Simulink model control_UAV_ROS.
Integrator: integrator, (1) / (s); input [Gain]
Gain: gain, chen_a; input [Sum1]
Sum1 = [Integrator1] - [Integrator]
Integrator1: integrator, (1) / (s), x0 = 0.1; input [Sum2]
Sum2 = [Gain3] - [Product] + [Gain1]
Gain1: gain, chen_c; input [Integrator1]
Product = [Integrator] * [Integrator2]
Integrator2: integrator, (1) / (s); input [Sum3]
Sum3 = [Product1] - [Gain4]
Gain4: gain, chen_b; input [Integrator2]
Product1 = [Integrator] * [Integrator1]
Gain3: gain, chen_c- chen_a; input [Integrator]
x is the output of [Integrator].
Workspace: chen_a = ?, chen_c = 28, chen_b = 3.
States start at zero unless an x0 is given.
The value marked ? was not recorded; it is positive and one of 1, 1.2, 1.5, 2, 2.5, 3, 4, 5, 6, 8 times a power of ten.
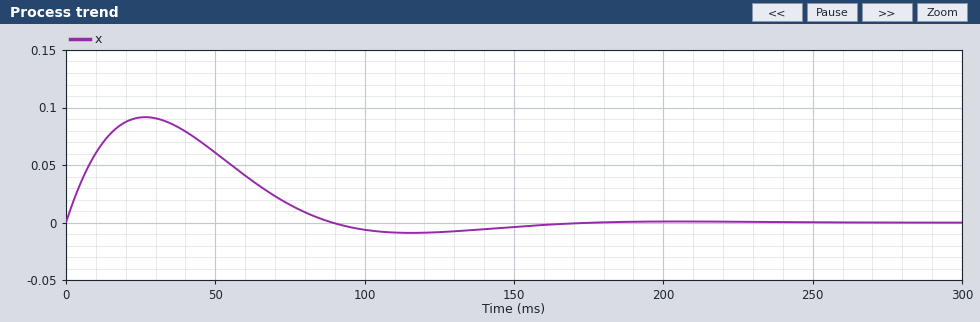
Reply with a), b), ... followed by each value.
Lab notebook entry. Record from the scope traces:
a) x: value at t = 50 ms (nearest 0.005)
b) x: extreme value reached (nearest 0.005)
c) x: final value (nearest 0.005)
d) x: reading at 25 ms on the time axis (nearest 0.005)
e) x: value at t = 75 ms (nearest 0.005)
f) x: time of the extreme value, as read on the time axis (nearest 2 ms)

a) 0.060
b) 0.090
c) 0.000
d) 0.090
e) 0.015
f) 26 ms
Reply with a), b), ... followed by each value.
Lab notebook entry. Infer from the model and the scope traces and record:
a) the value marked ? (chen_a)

a) 80
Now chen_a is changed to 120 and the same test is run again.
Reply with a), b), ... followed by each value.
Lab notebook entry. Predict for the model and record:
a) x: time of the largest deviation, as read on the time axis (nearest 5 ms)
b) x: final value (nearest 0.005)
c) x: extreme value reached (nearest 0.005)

a) 15 ms
b) 0.000
c) 0.075
